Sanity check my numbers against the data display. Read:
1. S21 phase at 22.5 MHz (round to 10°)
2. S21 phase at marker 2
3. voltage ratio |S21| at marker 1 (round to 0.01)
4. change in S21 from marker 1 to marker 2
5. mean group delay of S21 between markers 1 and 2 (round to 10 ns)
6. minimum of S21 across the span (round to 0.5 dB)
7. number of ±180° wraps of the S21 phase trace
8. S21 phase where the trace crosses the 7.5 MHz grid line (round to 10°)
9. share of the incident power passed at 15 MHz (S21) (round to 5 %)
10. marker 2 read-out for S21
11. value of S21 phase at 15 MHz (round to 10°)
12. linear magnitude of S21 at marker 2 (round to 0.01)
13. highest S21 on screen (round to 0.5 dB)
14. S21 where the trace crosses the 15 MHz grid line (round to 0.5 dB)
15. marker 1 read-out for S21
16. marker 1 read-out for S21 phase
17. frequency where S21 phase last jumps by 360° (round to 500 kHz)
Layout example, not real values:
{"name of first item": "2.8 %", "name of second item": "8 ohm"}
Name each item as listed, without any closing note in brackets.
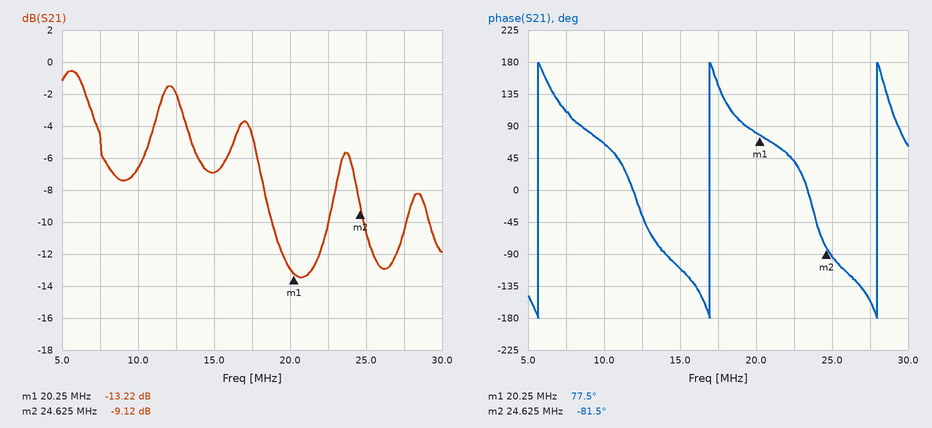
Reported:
{"S21 phase at 22.5 MHz": "40°", "S21 phase at marker 2": "-81.5°", "voltage ratio |S21| at marker 1": "0.22", "change in S21 from marker 1 to marker 2": "4.10 dB", "mean group delay of S21 between markers 1 and 2": "100 ns", "minimum of S21 across the span": "-13.5 dB", "number of ±180° wraps of the S21 phase trace": "3", "S21 phase where the trace crosses the 7.5 MHz grid line": "110°", "share of the incident power passed at 15 MHz (S21)": "20 %", "marker 2 read-out for S21": "-9.12 dB", "value of S21 phase at 15 MHz": "-110°", "linear magnitude of S21 at marker 2": "0.35", "highest S21 on screen": "-0.5 dB", "S21 where the trace crosses the 15 MHz grid line": "-7.0 dB", "marker 1 read-out for S21": "-13.22 dB", "marker 1 read-out for S21 phase": "77.5°", "frequency where S21 phase last jumps by 360°": "28.0 MHz"}
